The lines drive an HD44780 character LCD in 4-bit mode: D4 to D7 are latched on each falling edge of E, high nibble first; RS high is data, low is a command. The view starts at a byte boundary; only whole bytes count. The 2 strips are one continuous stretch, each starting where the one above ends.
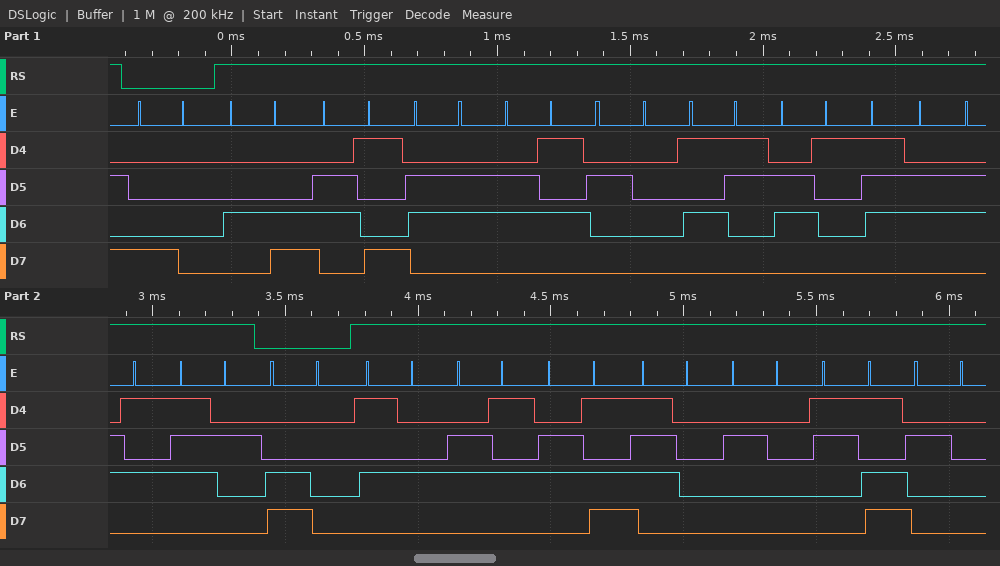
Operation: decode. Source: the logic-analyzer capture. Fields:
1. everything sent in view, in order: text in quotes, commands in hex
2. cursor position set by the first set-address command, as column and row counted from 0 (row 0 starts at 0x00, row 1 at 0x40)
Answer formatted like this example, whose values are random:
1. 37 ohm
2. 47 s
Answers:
1. 0x80 "Life Saver" 0xC0 "Temp = "
2. column 0, row 0
